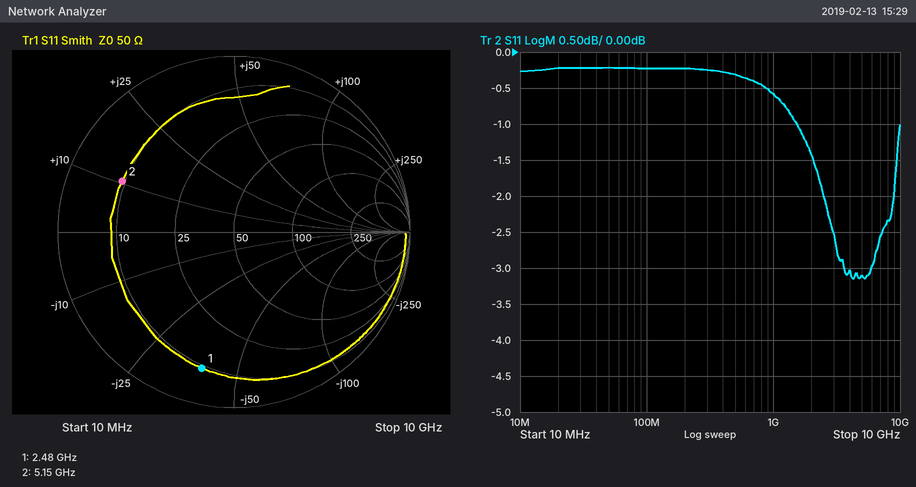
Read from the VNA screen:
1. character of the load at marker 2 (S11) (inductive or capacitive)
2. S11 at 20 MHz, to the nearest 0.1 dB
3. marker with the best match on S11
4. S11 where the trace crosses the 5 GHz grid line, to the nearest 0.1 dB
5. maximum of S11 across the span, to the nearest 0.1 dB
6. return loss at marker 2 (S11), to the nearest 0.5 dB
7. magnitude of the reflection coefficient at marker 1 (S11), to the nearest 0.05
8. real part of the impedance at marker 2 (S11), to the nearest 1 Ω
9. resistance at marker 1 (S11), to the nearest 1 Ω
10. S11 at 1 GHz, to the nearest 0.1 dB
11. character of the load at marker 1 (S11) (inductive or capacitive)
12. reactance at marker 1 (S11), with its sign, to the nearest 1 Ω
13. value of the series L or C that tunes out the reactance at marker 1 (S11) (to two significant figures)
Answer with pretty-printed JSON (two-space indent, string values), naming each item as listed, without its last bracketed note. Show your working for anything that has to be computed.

{
  "character of the load at marker 2 (S11)": "inductive",
  "S11 at 20 MHz, to the nearest 0.1 dB": "-0.2 dB",
  "marker with the best match on S11": "marker 2",
  "S11 where the trace crosses the 5 GHz grid line, to the nearest 0.1 dB": "-3.1 dB",
  "maximum of S11 across the span, to the nearest 0.1 dB": "-0.2 dB",
  "return loss at marker 2 (S11), to the nearest 0.5 dB": "3.0 dB",
  "magnitude of the reflection coefficient at marker 1 (S11), to the nearest 0.05": "0.80",
  "real part of the impedance at marker 2 (S11), to the nearest 1 Ω": "9 Ω",
  "resistance at marker 1 (S11), to the nearest 1 Ω": "9 Ω",
  "S11 at 1 GHz, to the nearest 0.1 dB": "-0.6 dB",
  "character of the load at marker 1 (S11)": "capacitive",
  "reactance at marker 1 (S11), with its sign, to the nearest 1 Ω": "-39 Ω",
  "value of the series L or C that tunes out the reactance at marker 1 (S11)": "L = 39 Ω/(2π × 2.48 GHz) ≈ 2.5 nH"
}
